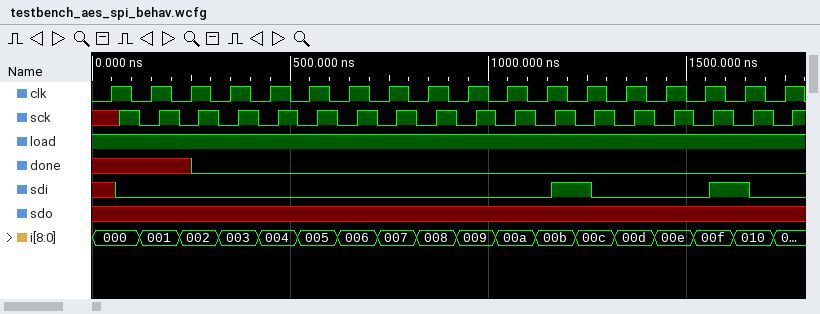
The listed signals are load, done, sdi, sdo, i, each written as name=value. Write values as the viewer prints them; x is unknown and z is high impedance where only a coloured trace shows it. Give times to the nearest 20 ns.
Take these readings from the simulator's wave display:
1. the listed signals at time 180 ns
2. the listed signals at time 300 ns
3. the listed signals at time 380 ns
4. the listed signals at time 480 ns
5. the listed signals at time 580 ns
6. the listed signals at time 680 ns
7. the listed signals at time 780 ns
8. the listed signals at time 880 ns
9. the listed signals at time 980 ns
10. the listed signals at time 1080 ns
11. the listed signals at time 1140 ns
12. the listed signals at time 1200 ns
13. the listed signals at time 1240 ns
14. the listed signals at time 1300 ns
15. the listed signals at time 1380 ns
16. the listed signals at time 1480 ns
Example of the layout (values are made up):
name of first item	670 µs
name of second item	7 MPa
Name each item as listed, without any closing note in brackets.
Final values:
the listed signals at time 180 ns	load=1, done=x, sdi=0, sdo=x, i=001
the listed signals at time 300 ns	load=1, done=0, sdi=0, sdo=x, i=002
the listed signals at time 380 ns	load=1, done=0, sdi=0, sdo=x, i=003
the listed signals at time 480 ns	load=1, done=0, sdi=0, sdo=x, i=004
the listed signals at time 580 ns	load=1, done=0, sdi=0, sdo=x, i=005
the listed signals at time 680 ns	load=1, done=0, sdi=0, sdo=x, i=006
the listed signals at time 780 ns	load=1, done=0, sdi=0, sdo=x, i=007
the listed signals at time 880 ns	load=1, done=0, sdi=0, sdo=x, i=008
the listed signals at time 980 ns	load=1, done=0, sdi=0, sdo=x, i=009
the listed signals at time 1080 ns	load=1, done=0, sdi=0, sdo=x, i=00a
the listed signals at time 1140 ns	load=1, done=0, sdi=0, sdo=x, i=00b
the listed signals at time 1200 ns	load=1, done=0, sdi=1, sdo=x, i=00b
the listed signals at time 1240 ns	load=1, done=0, sdi=1, sdo=x, i=00c
the listed signals at time 1300 ns	load=1, done=0, sdi=0, sdo=x, i=00c
the listed signals at time 1380 ns	load=1, done=0, sdi=0, sdo=x, i=00d
the listed signals at time 1480 ns	load=1, done=0, sdi=0, sdo=x, i=00e
